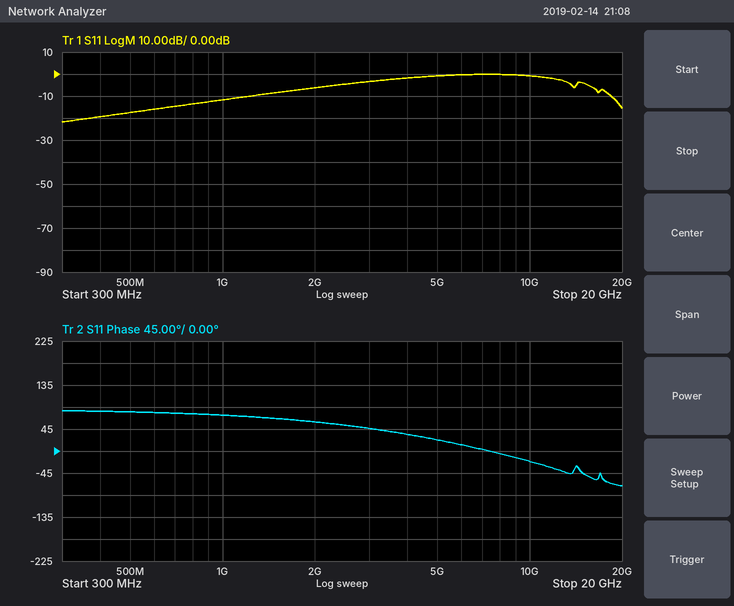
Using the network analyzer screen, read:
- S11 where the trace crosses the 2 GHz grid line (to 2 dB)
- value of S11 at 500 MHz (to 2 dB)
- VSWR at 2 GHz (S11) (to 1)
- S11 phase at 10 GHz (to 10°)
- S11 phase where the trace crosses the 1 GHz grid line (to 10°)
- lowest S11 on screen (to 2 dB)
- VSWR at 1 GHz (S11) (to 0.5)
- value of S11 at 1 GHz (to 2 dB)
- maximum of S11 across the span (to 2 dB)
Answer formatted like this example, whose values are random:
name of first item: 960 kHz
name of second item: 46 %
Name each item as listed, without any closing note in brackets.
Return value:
S11 where the trace crosses the 2 GHz grid line: -6 dB
value of S11 at 500 MHz: -18 dB
VSWR at 2 GHz (S11): 3
S11 phase at 10 GHz: -20°
S11 phase where the trace crosses the 1 GHz grid line: 70°
lowest S11 on screen: -22 dB
VSWR at 1 GHz (S11): 1.5
value of S11 at 1 GHz: -12 dB
maximum of S11 across the span: 0 dB
